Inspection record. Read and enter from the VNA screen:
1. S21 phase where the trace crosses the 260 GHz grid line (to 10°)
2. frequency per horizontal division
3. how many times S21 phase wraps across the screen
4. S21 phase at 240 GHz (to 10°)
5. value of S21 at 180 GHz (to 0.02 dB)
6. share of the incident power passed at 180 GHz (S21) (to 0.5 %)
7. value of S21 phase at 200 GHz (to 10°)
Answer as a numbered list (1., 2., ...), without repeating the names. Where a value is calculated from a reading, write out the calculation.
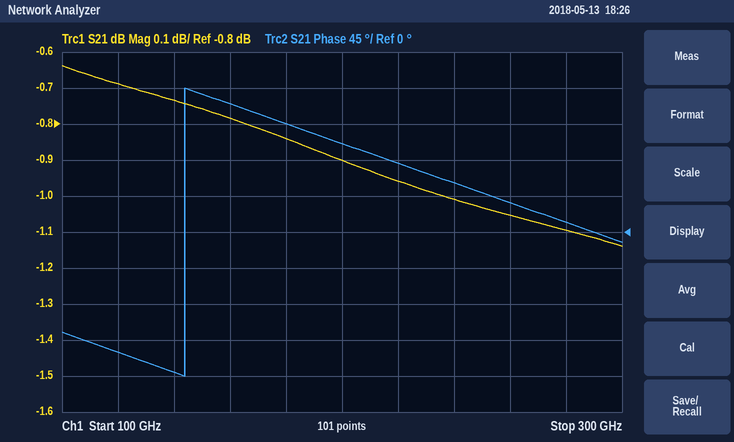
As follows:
1. 40°
2. 20 GHz
3. 1
4. 60°
5. -0.84 dB
6. 10^(-0.84/10) ≈ 82.4 %, so 82.5 % to the nearest 0.5 %
7. 110°
